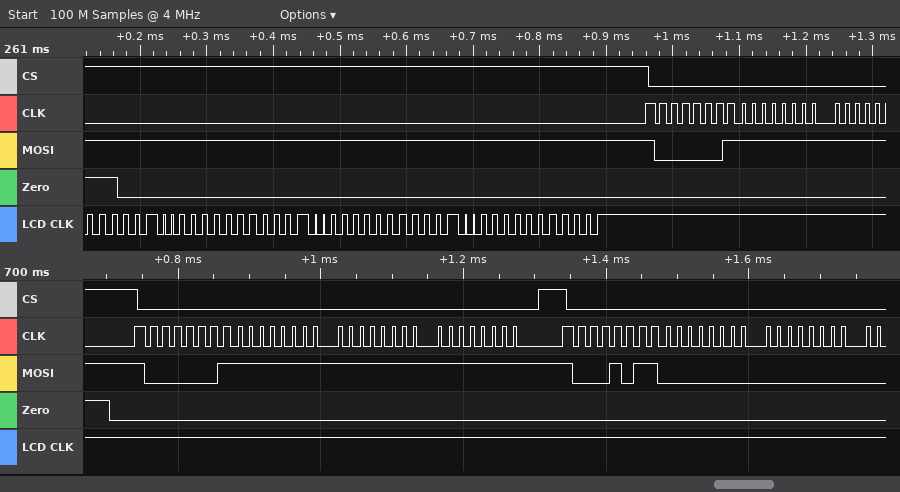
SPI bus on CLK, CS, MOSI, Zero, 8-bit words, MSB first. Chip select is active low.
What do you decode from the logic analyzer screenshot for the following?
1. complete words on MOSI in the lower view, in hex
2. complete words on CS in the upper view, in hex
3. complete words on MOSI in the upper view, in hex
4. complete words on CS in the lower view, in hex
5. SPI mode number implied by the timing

81, FF, FF, FF, 8B, 00, 00
80, 00
81, FF
80, 00, 00, 00, 80, 00, 00
0
